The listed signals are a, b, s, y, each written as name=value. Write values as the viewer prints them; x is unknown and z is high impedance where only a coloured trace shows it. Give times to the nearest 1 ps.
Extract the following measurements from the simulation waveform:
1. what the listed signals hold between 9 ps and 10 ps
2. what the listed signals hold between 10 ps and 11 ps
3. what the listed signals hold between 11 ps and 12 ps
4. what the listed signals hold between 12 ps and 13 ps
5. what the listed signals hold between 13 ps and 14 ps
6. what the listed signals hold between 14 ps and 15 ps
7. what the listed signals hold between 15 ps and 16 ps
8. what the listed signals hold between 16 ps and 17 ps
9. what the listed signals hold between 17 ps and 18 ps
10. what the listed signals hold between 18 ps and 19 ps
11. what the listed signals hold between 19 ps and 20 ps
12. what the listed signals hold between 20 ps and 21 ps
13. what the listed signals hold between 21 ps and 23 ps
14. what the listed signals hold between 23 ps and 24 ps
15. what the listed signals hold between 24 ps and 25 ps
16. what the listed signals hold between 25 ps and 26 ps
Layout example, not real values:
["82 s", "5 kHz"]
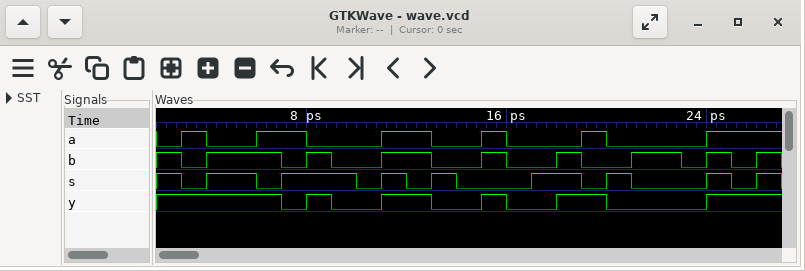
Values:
["a=0, b=0, s=1, y=0", "a=0, b=0, s=0, y=0", "a=1, b=1, s=1, y=1", "a=1, b=1, s=0, y=1", "a=0, b=0, s=1, y=0", "a=0, b=0, s=0, y=0", "a=1, b=1, s=0, y=1", "a=0, b=0, s=0, y=0", "a=0, b=0, s=1, y=0", "a=0, b=1, s=1, y=1", "a=1, b=0, s=0, y=1", "a=0, b=0, s=1, y=0", "a=0, b=1, s=0, y=0", "a=0, b=0, s=0, y=0", "a=1, b=1, s=1, y=1", "a=1, b=0, s=0, y=1"]
